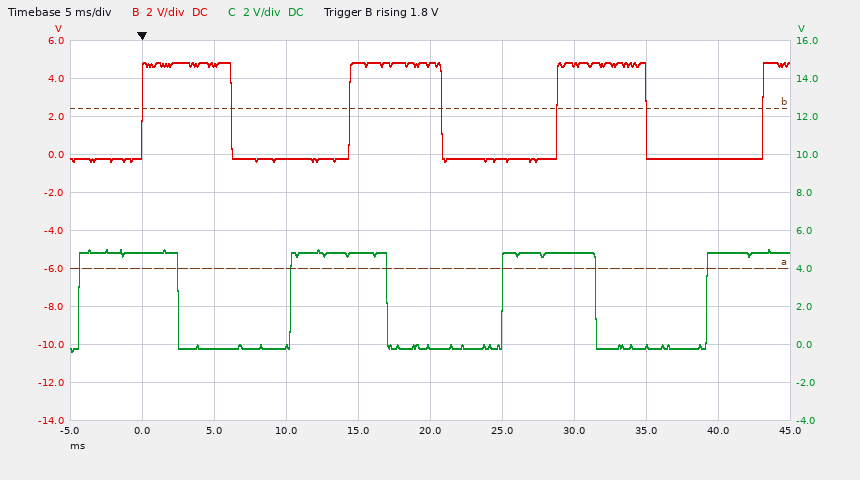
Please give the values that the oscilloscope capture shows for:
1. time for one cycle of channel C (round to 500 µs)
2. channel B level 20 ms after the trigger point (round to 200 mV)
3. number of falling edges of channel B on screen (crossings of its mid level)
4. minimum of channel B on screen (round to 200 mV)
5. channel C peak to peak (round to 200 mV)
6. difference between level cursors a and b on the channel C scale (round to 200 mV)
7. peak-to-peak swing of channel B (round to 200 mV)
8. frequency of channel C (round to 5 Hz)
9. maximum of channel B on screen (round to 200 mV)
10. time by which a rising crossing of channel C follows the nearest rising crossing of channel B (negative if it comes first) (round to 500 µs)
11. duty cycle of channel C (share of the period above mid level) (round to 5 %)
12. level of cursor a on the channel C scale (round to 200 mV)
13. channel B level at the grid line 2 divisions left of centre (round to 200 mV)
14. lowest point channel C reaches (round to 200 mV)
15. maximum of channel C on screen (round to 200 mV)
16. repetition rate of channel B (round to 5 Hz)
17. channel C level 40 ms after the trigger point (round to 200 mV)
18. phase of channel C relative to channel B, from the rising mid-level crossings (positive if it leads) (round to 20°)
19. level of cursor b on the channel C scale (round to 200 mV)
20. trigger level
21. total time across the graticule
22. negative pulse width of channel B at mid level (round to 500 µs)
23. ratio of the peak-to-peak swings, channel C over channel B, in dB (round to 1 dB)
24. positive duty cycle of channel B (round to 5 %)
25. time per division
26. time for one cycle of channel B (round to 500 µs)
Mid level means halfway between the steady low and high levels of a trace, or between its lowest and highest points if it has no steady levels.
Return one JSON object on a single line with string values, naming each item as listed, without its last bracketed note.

{"time for one cycle of channel C": "14.5 ms", "channel B level 20 ms after the trigger point": "4.8 V", "number of falling edges of channel B on screen": "3", "minimum of channel B on screen": "-400 mV", "channel C peak to peak": "5.4 V", "difference between level cursors a and b on the channel C scale": "8.4 V", "peak-to-peak swing of channel B": "5.2 V", "frequency of channel C": "70 Hz", "maximum of channel B on screen": "4.8 V", "time by which a rising crossing of channel C follows the nearest rising crossing of channel B (negative if it comes first)": "-4.0 ms", "duty cycle of channel C (share of the period above mid level)": "45 %", "level of cursor a on the channel C scale": "4.0 V", "channel B level at the grid line 2 divisions left of centre": "-200 mV", "lowest point channel C reaches": "-400 mV", "maximum of channel C on screen": "5.0 V", "repetition rate of channel B": "70 Hz", "channel C level 40 ms after the trigger point": "4.8 V", "phase of channel C relative to channel B, from the rising mid-level crossings (positive if it leads)": "+100°", "level of cursor b on the channel C scale": "12.4 V", "trigger level": "1.8 V", "total time across the graticule": "50 ms", "negative pulse width of channel B at mid level": "8.0 ms", "ratio of the peak-to-peak swings, channel C over channel B, in dB": "0 dB", "positive duty cycle of channel B": "45 %", "time per division": "5 ms", "time for one cycle of channel B": "14.5 ms"}
